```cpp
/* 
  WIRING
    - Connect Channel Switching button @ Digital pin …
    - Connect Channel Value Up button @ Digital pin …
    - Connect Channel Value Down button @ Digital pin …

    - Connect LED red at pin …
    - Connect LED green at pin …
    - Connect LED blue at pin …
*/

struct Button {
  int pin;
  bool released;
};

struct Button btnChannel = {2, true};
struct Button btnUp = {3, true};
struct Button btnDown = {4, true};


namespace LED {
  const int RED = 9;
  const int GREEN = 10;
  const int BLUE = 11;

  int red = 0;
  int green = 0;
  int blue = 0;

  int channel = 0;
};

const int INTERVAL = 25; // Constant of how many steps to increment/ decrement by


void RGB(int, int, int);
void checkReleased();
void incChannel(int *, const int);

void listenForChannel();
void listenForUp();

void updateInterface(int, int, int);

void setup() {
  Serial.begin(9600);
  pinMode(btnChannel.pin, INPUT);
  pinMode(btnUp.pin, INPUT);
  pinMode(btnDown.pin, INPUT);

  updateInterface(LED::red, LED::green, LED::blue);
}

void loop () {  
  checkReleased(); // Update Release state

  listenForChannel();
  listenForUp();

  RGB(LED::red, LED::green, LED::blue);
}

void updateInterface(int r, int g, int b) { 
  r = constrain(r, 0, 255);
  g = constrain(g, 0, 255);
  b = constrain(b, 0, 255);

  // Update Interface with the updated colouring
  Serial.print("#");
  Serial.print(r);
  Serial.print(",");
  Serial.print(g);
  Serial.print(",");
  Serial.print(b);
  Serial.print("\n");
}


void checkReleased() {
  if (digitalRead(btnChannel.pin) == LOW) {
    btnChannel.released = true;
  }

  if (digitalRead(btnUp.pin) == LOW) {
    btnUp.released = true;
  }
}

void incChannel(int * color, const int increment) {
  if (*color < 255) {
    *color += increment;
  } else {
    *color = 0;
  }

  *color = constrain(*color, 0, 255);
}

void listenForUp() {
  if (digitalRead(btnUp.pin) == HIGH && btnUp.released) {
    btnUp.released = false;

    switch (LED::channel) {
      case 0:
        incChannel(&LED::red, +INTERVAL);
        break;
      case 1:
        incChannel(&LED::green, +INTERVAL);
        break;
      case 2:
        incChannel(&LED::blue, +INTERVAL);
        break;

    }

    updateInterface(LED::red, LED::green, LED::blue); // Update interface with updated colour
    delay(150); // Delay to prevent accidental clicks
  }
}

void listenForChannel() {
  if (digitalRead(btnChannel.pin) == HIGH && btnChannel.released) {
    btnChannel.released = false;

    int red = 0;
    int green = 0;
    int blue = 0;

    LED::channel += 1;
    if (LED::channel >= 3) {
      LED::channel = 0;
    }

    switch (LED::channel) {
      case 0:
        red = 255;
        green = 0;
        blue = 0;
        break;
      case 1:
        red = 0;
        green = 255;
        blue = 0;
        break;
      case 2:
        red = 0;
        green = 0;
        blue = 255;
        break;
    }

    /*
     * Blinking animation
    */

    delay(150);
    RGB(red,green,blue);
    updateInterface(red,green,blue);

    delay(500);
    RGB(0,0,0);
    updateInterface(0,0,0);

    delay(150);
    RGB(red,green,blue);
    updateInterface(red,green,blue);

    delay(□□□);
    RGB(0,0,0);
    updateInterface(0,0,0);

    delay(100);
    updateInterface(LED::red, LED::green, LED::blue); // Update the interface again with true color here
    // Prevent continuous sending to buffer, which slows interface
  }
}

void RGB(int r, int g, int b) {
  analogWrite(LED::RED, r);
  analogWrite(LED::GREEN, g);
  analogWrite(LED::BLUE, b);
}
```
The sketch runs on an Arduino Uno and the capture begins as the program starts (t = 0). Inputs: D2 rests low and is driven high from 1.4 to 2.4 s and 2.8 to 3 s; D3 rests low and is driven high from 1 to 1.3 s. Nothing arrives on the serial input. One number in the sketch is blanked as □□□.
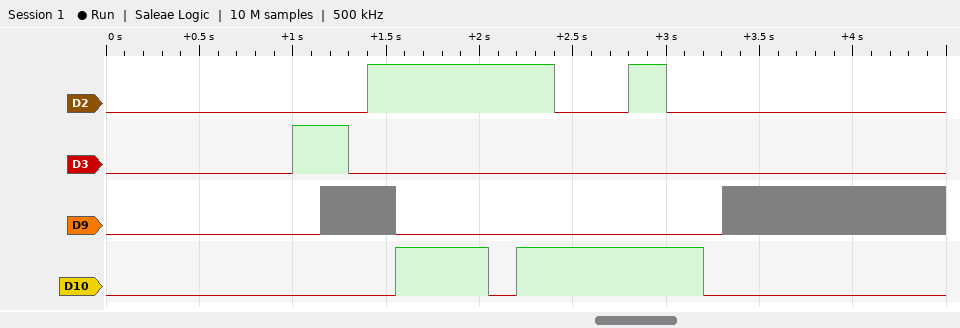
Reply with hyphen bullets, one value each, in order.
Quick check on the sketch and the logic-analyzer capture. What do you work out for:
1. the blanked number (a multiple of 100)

- 1000
